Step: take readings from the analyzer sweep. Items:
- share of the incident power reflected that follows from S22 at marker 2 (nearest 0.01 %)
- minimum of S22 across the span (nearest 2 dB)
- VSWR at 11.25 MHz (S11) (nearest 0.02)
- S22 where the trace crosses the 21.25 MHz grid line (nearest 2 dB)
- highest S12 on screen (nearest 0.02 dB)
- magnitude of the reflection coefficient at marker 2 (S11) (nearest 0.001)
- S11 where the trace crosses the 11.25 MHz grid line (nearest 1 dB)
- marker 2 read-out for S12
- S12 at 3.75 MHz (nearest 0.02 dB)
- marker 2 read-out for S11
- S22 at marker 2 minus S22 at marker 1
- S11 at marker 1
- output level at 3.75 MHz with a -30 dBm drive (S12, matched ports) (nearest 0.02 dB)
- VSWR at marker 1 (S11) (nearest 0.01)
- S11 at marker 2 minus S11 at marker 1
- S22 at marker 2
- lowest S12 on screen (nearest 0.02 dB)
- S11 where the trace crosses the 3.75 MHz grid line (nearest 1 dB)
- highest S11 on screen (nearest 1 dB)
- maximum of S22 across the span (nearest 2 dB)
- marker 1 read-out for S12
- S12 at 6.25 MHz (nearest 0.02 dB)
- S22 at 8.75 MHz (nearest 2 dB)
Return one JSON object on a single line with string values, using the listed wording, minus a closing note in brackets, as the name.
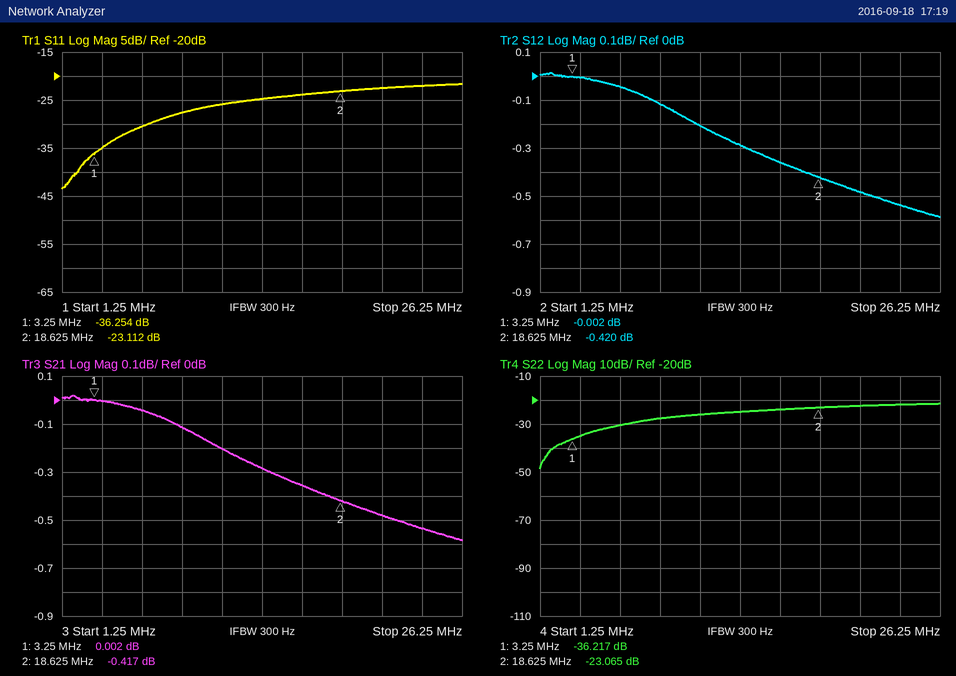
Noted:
{"share of the incident power reflected that follows from S22 at marker 2": "0.49 %", "minimum of S22 across the span": "-48 dB", "VSWR at 11.25 MHz (S11)": "1.10", "S22 where the trace crosses the 21.25 MHz grid line": "-22 dB", "highest S12 on screen": "0.02 dB", "magnitude of the reflection coefficient at marker 2 (S11)": "0.070", "S11 where the trace crosses the 11.25 MHz grid line": "-26 dB", "marker 2 read-out for S12": "-0.420 dB", "S12 at 3.75 MHz": "0.00 dB", "marker 2 read-out for S11": "-23.112 dB", "S22 at marker 2 minus S22 at marker 1": "13.152 dB", "S11 at marker 1": "-36.254 dB", "output level at 3.75 MHz with a -30 dBm drive (S12, matched ports)": "-30.00 dBm", "VSWR at marker 1 (S11)": "1.03", "S11 at marker 2 minus S11 at marker 1": "13.142 dB", "S22 at marker 2": "-23.065 dB", "lowest S12 on screen": "-0.58 dB", "S11 where the trace crosses the 3.75 MHz grid line": "-35 dB", "highest S11 on screen": "-22 dB", "maximum of S22 across the span": "-22 dB", "marker 1 read-out for S12": "-0.002 dB", "S12 at 6.25 MHz": "-0.04 dB", "S22 at 8.75 MHz": "-28 dB"}
